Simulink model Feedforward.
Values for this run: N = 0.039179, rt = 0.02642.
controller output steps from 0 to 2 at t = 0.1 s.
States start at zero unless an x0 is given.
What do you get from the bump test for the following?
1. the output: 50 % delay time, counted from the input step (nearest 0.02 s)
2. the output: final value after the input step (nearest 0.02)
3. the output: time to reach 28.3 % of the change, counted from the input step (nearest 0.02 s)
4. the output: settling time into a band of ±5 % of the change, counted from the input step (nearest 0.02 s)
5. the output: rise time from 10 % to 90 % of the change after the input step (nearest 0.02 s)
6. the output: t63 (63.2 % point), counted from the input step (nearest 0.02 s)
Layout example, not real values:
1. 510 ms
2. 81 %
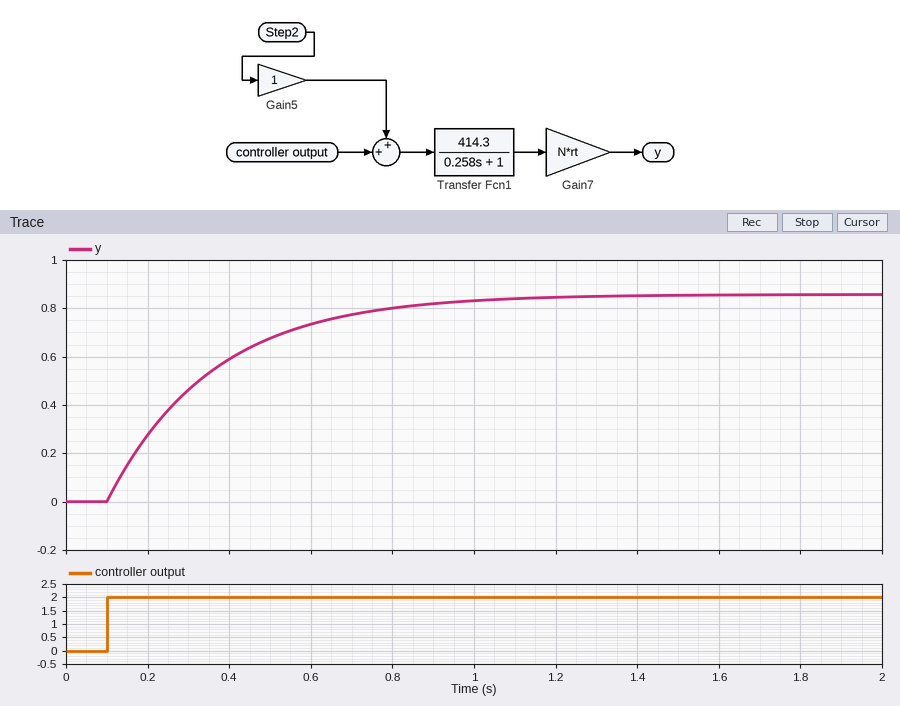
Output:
1. 0.18 s
2. 0.86
3. 0.08 s
4. 0.78 s
5. 0.56 s
6. 0.26 s
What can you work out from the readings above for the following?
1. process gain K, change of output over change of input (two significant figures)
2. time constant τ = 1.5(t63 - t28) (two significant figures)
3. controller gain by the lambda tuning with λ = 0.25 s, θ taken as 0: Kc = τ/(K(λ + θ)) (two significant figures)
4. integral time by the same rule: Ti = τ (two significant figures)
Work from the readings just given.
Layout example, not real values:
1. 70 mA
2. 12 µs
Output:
1. 0.43
2. 0.27 s
3. 2.5
4. 0.27 s
